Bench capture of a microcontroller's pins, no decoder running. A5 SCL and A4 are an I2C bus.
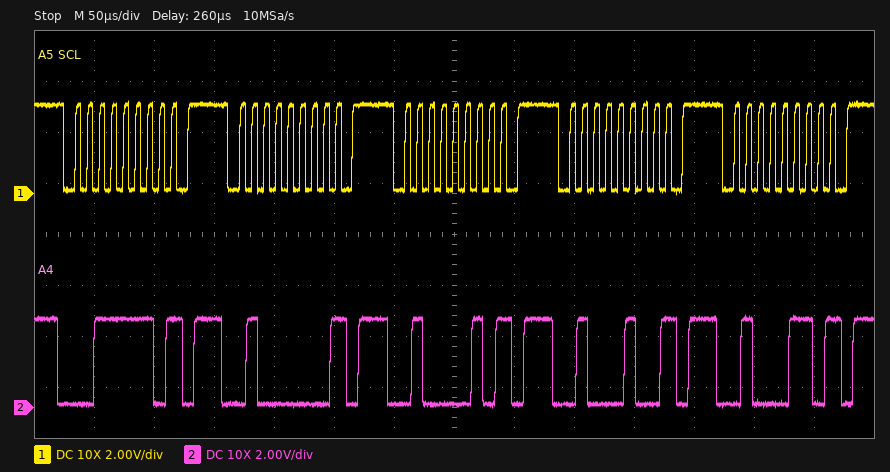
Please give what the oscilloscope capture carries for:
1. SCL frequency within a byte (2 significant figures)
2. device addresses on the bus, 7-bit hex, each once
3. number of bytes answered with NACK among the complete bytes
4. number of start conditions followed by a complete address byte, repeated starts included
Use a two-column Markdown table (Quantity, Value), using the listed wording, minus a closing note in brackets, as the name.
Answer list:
| Quantity | Value |
|---|---|
| SCL frequency within a byte | 100 kHz |
| device addresses on the bus, 7-bit hex, each once | 0x1F 0x20 0x21 0x22 0x23 |
| number of bytes answered with NACK among the complete bytes | 5 |
| number of start conditions followed by a complete address byte, repeated starts included | 5 |
